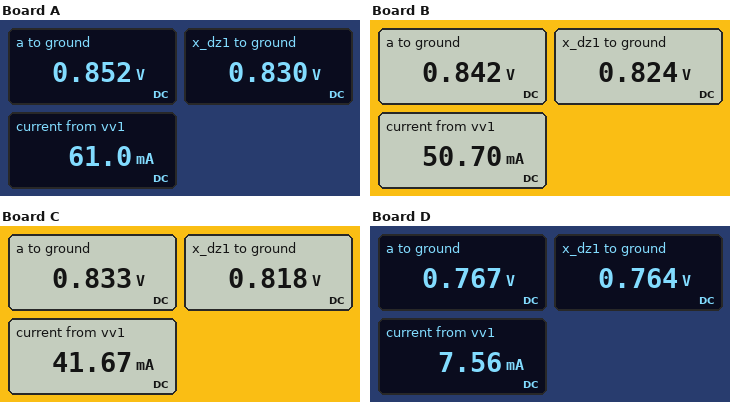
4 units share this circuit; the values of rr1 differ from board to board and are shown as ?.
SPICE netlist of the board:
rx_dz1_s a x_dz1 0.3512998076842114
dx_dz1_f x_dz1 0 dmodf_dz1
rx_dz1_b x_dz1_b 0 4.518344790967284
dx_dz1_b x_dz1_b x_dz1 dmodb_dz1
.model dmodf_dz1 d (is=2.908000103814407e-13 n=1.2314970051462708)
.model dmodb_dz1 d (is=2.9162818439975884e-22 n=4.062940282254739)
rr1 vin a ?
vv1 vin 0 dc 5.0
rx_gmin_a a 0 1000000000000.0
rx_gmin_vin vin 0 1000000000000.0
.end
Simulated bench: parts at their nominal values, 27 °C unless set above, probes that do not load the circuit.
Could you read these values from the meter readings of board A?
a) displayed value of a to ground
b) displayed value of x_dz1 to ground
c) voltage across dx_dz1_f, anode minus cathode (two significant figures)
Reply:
0.852 V
0.830 V
830 mV
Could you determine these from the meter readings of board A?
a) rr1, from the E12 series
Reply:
68 Ω
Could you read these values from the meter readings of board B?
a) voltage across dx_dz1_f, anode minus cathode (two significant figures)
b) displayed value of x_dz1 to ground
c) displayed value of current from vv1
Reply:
820 mV
0.824 V
50.70 mA
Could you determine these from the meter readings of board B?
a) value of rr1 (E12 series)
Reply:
82 Ω
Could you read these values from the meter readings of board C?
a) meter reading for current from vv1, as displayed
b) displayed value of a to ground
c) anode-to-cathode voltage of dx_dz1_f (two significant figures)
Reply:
41.67 mA
0.833 V
820 mV
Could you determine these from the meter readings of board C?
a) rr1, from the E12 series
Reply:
100 Ω
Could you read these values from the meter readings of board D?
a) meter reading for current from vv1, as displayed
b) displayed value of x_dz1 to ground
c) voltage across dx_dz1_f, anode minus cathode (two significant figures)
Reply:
7.56 mA
0.764 V
760 mV
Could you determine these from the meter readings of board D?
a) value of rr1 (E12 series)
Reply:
560 Ω
